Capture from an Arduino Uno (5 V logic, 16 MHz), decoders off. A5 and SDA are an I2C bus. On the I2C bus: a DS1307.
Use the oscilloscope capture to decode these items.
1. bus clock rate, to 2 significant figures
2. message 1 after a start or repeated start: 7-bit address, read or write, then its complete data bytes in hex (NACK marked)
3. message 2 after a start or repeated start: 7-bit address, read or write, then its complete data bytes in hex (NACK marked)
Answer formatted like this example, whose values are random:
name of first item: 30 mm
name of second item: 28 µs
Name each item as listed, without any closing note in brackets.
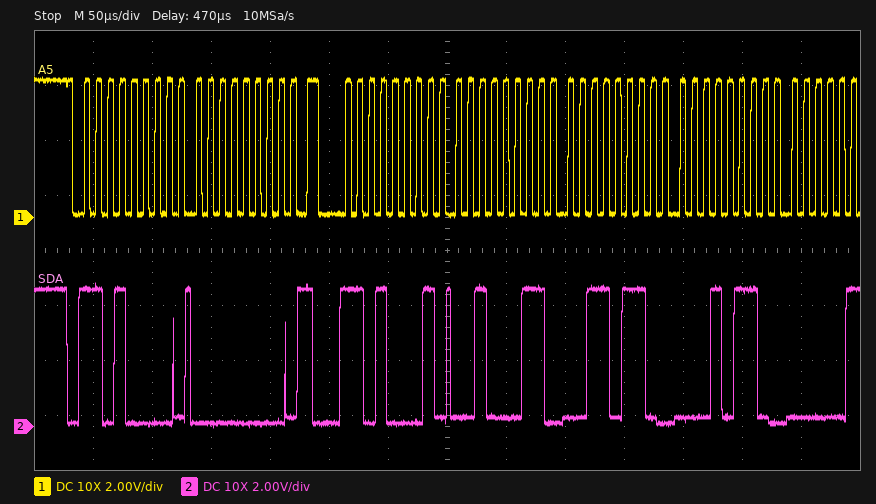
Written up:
bus clock rate, to 2 significant figures: 100 kHz
message 1 after a start or repeated start: 7-bit address, read or write, then its complete data bytes in hex: 0x68 write: 00
message 2 after a start or repeated start: 7-bit address, read or write, then its complete data bytes in hex: 0x68 read: 23 36 16
